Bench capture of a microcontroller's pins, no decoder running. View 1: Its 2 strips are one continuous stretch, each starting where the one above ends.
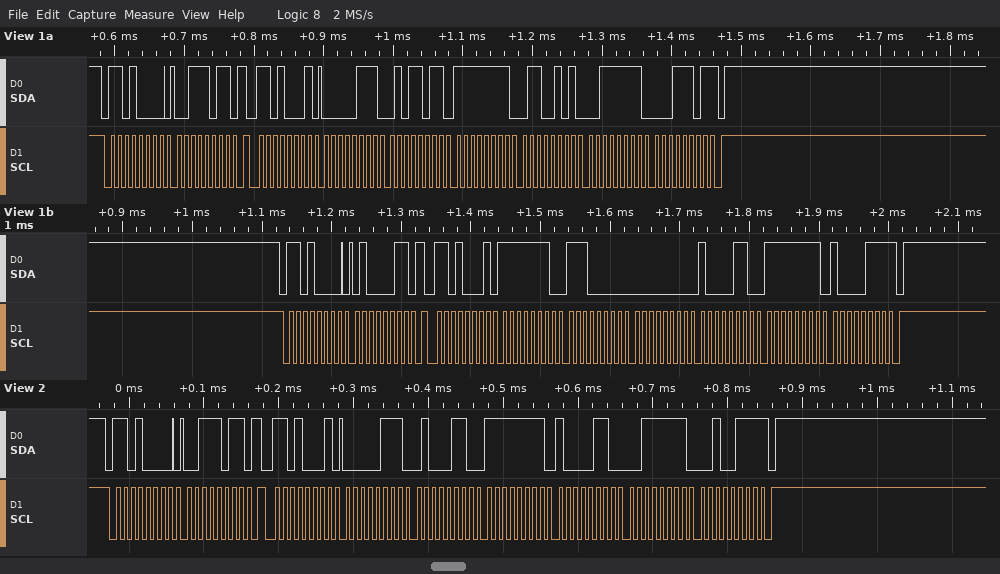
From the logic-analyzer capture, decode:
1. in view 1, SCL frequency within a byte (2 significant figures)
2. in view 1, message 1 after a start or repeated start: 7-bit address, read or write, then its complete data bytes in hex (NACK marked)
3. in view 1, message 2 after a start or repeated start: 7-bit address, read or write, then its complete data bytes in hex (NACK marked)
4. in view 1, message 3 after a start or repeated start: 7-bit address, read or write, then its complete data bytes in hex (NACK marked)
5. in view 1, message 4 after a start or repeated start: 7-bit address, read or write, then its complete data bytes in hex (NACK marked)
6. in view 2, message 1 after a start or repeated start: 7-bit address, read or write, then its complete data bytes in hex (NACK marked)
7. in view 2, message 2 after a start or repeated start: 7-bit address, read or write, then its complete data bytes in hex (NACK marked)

100 kHz
0x68 write: 3B
0x68 read: 07 5B FF 65 3F 1D NACK
0x68 write: 43
0x68 read: FE E0 00 86 FF 87 NACK
0x68 write: 3B
0x68 read: 07 46 FF 86 3F 27 NACK
